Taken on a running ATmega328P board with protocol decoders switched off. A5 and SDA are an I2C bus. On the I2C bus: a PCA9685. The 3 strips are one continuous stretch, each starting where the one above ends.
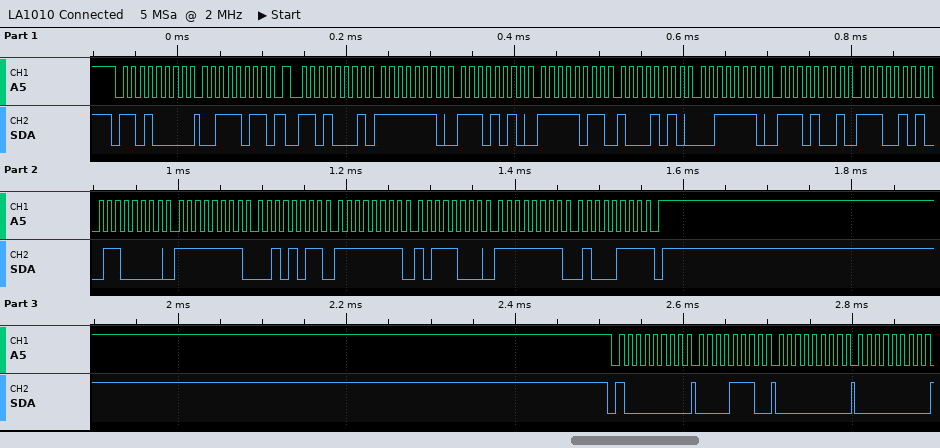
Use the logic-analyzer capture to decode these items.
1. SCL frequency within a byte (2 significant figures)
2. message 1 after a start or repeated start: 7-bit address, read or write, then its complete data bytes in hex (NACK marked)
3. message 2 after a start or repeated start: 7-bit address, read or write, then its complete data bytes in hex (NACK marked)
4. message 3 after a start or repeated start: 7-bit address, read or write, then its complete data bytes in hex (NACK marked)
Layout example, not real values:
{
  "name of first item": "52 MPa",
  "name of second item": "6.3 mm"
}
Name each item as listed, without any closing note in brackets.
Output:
{
  "SCL frequency within a byte": "100 kHz",
  "message 1 after a start or repeated start: 7-bit address, read or write, then its complete data bytes in hex": "0x68 write: 3B",
  "message 2 after a start or repeated start: 7-bit address, read or write, then its complete data bytes in hex": "0x68 read: FE EA FB 8A 3E E9 E5 60 FF 2B FF B8 FF 47 NACK",
  "message 3 after a start or repeated start: 7-bit address, read or write, then its complete data bytes in hex": "0x40 write: 0E 00 00"
}
